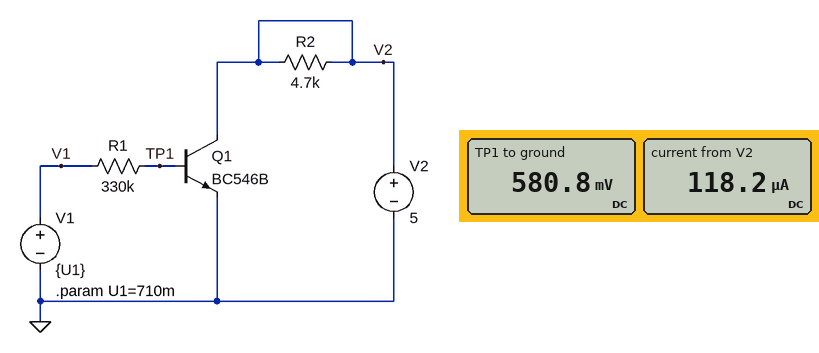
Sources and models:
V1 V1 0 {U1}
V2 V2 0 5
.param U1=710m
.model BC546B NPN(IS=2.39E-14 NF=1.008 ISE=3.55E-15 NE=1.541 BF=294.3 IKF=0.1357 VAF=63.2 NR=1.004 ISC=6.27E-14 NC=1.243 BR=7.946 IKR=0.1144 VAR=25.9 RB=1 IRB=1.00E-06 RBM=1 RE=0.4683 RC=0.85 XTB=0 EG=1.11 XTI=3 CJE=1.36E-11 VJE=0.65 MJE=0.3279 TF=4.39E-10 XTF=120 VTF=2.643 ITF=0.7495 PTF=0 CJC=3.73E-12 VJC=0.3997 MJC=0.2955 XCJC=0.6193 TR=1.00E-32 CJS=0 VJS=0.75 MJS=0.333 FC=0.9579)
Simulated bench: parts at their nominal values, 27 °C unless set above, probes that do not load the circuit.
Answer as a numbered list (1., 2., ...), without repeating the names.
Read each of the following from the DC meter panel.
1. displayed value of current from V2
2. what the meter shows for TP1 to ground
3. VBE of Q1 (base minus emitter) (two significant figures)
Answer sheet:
1. 118.2 µA
2. 580.8 mV
3. 580 mV
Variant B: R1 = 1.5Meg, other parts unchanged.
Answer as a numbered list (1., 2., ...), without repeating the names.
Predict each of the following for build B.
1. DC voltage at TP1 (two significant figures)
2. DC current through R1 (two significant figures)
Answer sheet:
1. 550 mV
2. 110 nA
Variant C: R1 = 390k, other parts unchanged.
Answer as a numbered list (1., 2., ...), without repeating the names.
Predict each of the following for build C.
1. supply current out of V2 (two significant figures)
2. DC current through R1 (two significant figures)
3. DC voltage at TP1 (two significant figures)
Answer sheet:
1. 100 µA
2. 340 nA
3. 580 mV
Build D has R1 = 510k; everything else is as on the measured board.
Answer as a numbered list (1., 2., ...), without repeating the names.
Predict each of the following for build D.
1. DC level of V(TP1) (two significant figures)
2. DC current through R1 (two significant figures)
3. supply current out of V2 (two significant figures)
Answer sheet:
1. 570 mV
2. 270 nA
3. 82 µA
